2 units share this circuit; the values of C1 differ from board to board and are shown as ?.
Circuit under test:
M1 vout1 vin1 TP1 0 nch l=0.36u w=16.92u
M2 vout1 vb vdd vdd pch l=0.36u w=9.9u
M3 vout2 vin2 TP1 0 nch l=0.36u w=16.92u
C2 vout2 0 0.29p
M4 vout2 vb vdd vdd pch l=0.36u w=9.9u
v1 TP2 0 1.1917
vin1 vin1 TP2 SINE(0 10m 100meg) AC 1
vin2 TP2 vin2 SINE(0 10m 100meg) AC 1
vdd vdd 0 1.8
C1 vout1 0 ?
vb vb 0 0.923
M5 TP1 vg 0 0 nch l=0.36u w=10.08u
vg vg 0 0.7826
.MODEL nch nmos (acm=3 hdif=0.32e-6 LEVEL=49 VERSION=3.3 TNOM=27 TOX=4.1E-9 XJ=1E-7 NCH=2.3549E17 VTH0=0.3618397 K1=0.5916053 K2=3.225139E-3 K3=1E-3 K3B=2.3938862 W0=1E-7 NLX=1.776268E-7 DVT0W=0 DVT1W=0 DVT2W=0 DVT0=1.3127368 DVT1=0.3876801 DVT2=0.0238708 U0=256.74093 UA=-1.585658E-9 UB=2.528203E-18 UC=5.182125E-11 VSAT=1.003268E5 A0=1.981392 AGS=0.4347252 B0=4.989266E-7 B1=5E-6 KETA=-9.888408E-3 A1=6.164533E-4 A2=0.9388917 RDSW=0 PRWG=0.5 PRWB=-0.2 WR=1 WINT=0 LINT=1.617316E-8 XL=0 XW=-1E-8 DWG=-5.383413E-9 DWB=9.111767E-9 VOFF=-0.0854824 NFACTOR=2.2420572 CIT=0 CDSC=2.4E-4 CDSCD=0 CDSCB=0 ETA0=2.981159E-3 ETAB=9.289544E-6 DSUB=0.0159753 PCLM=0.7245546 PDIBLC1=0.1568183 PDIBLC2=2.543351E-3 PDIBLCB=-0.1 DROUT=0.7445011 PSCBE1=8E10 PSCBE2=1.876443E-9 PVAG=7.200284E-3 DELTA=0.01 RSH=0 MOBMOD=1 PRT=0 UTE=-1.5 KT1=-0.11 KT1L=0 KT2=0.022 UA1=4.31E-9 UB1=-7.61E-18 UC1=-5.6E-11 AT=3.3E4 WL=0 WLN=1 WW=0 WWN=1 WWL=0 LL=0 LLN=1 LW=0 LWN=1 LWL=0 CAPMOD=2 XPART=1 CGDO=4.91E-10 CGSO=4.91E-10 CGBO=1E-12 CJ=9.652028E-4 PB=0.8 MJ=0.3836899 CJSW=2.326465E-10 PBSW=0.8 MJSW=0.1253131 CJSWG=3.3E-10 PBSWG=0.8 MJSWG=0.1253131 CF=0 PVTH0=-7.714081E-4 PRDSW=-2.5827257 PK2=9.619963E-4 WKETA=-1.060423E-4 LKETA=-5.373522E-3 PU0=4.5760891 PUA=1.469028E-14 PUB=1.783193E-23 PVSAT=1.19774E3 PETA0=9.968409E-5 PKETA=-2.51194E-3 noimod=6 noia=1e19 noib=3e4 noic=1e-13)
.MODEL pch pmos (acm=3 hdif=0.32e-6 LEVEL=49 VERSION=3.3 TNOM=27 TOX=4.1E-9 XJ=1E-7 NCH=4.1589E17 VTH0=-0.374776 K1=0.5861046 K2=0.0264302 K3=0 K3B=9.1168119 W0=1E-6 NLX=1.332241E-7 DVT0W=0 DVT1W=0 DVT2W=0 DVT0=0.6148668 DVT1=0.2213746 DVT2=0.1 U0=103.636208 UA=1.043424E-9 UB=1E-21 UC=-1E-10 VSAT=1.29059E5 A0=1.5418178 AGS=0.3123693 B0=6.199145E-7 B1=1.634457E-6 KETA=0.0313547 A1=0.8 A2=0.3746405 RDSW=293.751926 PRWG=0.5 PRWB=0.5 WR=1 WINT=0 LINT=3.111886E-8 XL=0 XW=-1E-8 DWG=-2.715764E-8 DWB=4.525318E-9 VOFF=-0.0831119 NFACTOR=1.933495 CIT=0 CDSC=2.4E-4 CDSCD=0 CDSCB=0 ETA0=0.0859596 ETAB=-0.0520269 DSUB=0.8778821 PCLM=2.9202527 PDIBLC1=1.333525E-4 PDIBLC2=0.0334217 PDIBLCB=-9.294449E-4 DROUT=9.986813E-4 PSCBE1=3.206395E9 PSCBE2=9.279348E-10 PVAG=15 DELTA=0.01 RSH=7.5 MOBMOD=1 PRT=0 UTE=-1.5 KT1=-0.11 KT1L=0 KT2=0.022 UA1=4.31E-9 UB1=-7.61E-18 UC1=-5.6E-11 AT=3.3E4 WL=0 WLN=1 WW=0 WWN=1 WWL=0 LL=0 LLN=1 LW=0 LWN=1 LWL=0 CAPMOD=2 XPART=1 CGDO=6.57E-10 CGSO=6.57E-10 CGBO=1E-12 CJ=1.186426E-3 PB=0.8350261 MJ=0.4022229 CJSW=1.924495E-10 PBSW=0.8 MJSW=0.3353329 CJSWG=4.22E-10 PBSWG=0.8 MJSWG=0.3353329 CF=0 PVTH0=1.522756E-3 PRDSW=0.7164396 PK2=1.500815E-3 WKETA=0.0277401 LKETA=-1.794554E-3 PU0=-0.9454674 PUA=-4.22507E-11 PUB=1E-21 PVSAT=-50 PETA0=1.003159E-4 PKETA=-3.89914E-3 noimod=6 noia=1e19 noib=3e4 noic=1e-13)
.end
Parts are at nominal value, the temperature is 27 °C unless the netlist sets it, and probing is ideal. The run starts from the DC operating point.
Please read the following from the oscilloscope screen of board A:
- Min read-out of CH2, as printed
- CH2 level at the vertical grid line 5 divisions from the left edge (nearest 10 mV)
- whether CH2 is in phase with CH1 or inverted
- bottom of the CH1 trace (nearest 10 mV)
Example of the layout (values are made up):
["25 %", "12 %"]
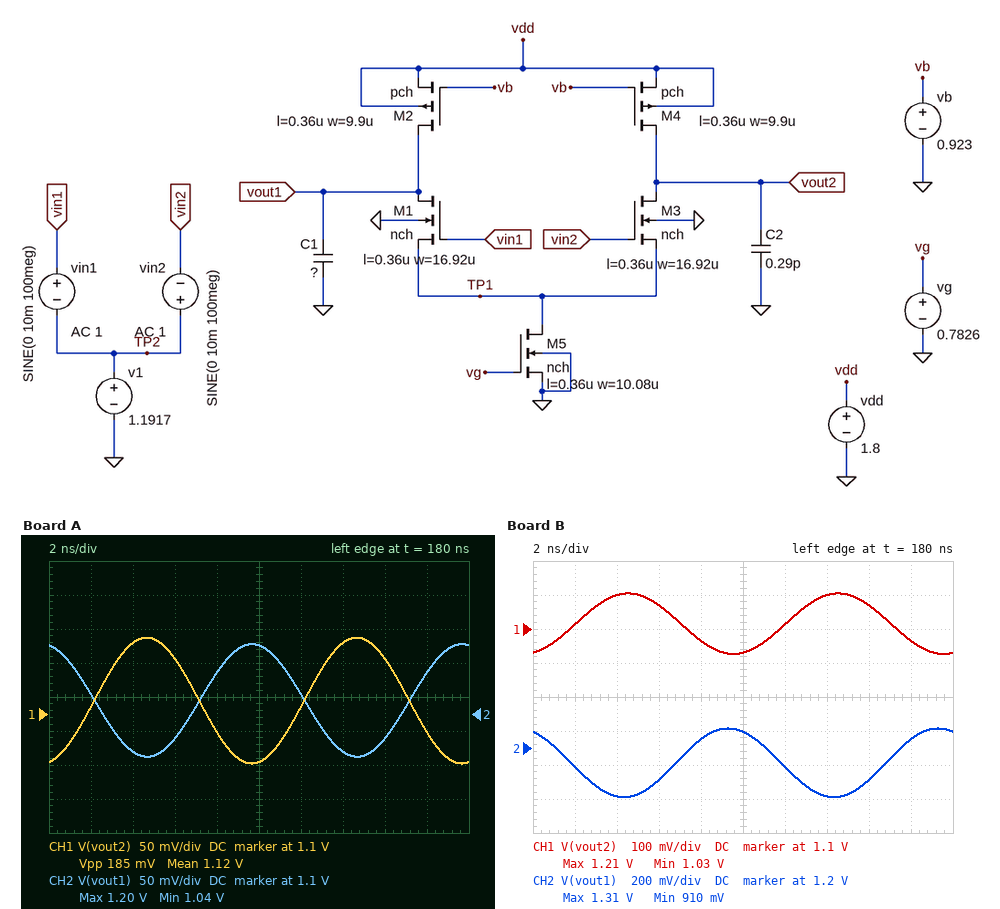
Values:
["1.04 V", "1.20 V", "inverted", "1.03 V"]
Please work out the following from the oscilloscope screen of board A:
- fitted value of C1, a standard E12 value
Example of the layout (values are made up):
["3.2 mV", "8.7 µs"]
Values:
["330 fF"]
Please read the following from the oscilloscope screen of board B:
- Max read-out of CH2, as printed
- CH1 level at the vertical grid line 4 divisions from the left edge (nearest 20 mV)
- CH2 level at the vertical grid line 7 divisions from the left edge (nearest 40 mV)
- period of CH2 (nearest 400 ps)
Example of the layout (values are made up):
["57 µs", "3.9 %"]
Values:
["1.31 V", "1.06 V", "920 mV", "10.0 ns"]
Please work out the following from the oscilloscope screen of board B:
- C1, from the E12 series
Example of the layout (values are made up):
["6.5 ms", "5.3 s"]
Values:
["100 fF"]
